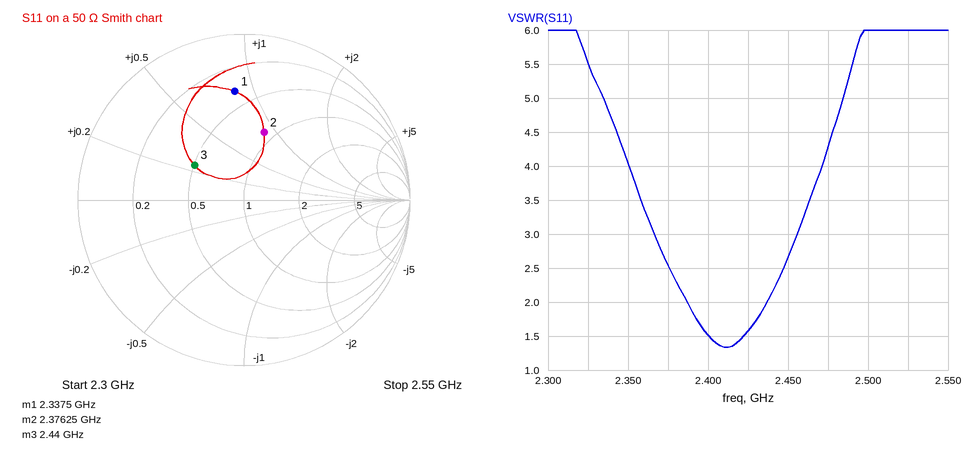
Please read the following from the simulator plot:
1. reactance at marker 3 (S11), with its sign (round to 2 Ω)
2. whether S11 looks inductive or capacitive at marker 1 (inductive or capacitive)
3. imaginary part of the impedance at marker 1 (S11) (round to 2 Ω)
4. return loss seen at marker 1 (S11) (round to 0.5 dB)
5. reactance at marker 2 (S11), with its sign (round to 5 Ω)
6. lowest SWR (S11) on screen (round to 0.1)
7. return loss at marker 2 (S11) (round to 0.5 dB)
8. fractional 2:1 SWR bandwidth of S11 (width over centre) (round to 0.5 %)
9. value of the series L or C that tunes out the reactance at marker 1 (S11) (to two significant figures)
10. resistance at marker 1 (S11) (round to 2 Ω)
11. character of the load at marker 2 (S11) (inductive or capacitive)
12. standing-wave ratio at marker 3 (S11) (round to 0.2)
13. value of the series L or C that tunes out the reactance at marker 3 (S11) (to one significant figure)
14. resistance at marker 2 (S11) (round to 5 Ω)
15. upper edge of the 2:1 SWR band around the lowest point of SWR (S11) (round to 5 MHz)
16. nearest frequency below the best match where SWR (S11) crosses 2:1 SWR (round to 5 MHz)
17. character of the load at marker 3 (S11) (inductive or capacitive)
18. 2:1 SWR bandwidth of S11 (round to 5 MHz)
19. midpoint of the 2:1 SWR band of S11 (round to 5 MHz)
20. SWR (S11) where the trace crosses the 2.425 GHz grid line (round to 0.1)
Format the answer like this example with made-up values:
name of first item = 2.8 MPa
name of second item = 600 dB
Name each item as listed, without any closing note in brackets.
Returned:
reactance at marker 3 (S11), with its sign = +12 Ω
whether S11 looks inductive or capacitive at marker 1 = inductive
imaginary part of the impedance at marker 1 (S11) = +42 Ω
return loss seen at marker 1 (S11) = 3.5 dB
reactance at marker 2 (S11), with its sign = +45 Ω
lowest SWR (S11) on screen = 1.3
return loss at marker 2 (S11) = 7.5 dB
fractional 2:1 SWR bandwidth of S11 (width over centre) = 2.0 %
value of the series L or C that tunes out the reactance at marker 1 (S11) = 1.6 pF
resistance at marker 1 (S11) = 18 Ω
character of the load at marker 2 (S11) = inductive
standing-wave ratio at marker 3 (S11) = 2.2
value of the series L or C that tunes out the reactance at marker 3 (S11) = 5 pF
resistance at marker 2 (S11) = 45 Ω
upper edge of the 2:1 SWR band around the lowest point of SWR (S11) = 2.435 GHz
nearest frequency below the best match where SWR (S11) crosses 2:1 SWR = 2.385 GHz
character of the load at marker 3 (S11) = inductive
2:1 SWR bandwidth of S11 = 50 MHz
midpoint of the 2:1 SWR band of S11 = 2.410 GHz
SWR (S11) where the trace crosses the 2.425 GHz grid line = 1.6
